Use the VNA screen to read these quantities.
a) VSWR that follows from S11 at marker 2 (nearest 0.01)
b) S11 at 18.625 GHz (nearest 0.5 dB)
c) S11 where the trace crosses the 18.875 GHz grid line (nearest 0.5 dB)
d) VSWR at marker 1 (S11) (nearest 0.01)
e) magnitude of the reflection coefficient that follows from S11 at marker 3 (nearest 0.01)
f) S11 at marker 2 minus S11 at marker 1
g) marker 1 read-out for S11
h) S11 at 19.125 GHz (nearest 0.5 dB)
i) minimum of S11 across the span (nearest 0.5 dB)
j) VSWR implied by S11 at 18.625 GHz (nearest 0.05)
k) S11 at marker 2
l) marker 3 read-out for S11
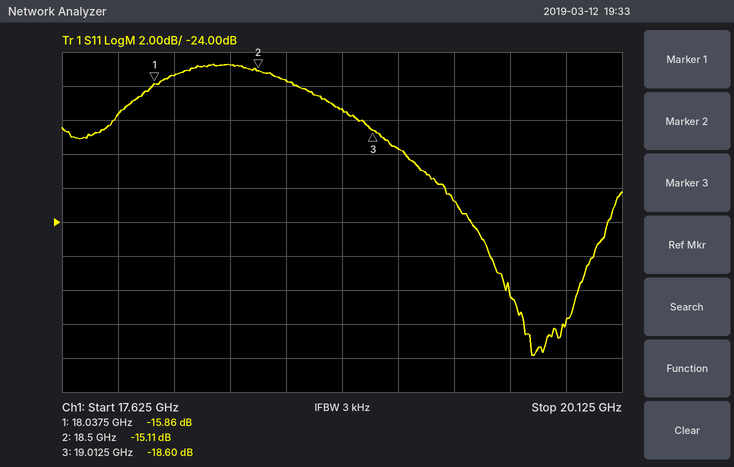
1.43
-15.5 dB
-17.5 dB
1.38
0.12
0.75 dB
-15.86 dB
-19.5 dB
-32.0 dB
1.40
-15.11 dB
-18.60 dB
